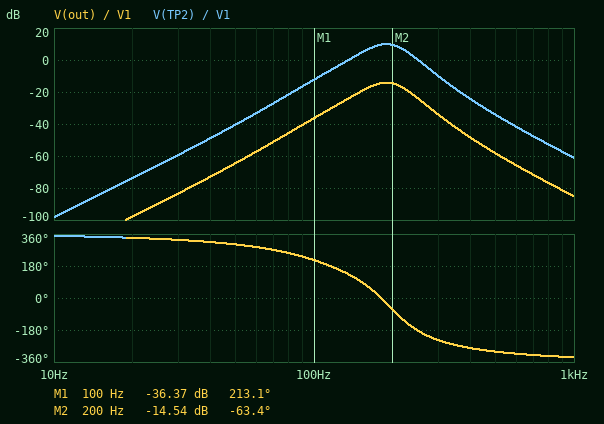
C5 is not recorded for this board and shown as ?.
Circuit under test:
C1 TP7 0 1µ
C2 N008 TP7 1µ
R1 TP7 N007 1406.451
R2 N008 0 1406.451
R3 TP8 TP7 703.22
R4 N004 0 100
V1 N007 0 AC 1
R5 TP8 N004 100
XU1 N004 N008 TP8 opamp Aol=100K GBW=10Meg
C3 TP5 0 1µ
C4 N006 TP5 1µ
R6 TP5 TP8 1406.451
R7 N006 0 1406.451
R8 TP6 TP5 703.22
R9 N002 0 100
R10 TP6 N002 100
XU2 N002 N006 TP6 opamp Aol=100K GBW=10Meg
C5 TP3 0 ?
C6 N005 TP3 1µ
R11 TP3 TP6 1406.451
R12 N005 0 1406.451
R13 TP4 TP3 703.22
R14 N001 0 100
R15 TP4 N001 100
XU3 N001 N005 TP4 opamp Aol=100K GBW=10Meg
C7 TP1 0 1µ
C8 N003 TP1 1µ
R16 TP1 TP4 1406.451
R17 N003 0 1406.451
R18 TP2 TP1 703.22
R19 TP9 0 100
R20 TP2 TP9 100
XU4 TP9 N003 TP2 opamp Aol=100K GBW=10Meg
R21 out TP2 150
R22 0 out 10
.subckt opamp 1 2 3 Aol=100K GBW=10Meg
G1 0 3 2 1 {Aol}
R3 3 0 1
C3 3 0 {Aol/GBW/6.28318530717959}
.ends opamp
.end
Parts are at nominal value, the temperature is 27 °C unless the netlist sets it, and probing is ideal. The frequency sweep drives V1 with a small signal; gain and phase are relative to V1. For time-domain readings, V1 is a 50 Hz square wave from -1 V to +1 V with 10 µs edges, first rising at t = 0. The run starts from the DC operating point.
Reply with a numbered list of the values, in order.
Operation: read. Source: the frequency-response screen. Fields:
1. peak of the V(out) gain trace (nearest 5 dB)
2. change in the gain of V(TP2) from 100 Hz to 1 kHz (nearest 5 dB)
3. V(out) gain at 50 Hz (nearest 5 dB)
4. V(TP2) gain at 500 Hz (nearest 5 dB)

1. -15 dB
2. -50 dB
3. -65 dB
4. -35 dB
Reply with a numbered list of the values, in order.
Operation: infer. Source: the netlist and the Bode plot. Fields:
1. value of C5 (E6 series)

1. 3.3 µF
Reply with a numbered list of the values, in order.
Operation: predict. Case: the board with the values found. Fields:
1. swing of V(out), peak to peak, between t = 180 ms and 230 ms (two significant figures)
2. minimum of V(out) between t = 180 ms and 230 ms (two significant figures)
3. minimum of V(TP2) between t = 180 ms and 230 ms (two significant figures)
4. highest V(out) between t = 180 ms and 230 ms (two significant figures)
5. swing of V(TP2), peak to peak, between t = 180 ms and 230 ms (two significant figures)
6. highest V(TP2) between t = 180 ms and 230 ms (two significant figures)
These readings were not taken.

1. 110 mV
2. -56 mV
3. -900 mV
4. 56 mV
5. 1.8 V
6. 900 mV
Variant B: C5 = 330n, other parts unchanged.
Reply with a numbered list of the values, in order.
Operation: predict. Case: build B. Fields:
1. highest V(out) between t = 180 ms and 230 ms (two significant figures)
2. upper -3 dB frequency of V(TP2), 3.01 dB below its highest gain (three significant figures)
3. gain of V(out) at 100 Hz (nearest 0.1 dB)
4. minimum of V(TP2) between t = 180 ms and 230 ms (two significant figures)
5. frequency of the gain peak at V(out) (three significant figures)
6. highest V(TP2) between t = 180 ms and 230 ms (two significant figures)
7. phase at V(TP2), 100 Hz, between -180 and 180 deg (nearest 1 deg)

1. 240 mV
2. 251 Hz
3. -35.8 dB
4. -3.8 V
5. 207 Hz
6. 3.8 V
7. -71 deg
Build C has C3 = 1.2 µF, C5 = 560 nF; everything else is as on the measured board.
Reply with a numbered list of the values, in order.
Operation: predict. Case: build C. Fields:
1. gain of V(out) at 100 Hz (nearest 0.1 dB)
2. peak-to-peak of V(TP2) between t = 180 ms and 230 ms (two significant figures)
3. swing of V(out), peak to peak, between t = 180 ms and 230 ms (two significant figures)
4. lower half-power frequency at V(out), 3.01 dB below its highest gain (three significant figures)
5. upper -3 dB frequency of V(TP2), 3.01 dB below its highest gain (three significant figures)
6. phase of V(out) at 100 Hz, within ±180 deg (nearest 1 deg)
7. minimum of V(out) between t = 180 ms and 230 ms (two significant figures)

1. -35.1 dB
2. 7.6 V
3. 470 mV
4. 177 Hz
5. 245 Hz
6. -82 deg
7. -240 mV
